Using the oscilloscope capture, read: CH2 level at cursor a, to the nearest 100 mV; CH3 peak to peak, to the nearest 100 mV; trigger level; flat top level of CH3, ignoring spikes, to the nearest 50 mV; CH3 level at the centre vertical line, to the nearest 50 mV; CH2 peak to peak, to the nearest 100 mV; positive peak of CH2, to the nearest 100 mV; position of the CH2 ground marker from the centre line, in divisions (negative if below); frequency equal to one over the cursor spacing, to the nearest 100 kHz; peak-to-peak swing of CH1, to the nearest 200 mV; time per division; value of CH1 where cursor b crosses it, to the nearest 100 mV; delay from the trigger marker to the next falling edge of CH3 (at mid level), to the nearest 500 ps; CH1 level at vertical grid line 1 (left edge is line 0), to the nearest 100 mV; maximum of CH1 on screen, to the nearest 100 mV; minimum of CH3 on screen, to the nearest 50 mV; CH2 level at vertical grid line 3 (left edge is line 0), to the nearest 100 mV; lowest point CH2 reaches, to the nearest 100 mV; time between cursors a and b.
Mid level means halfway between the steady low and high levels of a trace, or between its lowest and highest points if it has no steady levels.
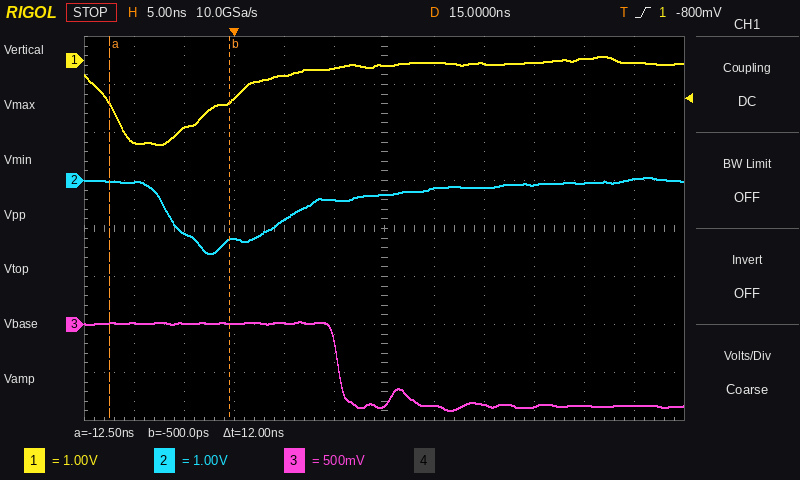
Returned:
0.0 V
900 mV
-800 mV
0 mV
-850 mV
1.6 V
100 mV
+1.0 div
83.3 MHz
1.8 V
5 ns
-900 mV
10.5 ns
-1.7 V
100 mV
-900 mV
-1.2 V
-1.5 V
12 ns
